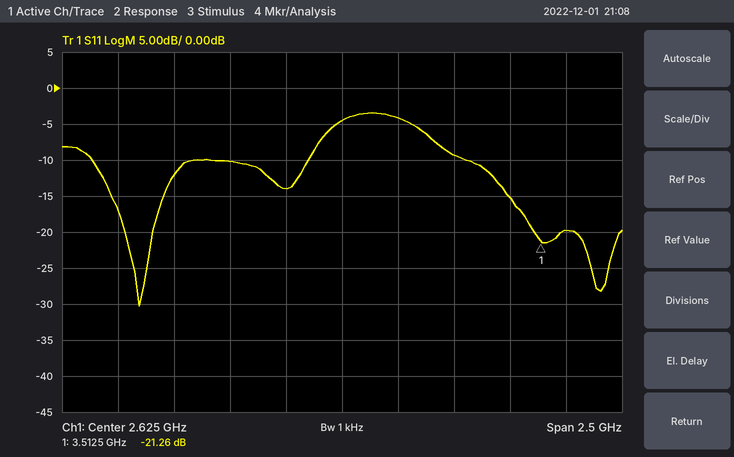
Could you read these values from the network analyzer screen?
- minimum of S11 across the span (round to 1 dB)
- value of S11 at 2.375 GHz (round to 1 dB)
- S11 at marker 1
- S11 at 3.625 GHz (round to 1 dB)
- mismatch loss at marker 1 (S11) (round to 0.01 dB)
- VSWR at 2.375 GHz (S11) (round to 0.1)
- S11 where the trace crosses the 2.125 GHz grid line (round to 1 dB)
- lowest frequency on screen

-30 dB
-14 dB
-21.26 dB
-20 dB
0.03 dB
1.5
-10 dB
1.375 GHz
